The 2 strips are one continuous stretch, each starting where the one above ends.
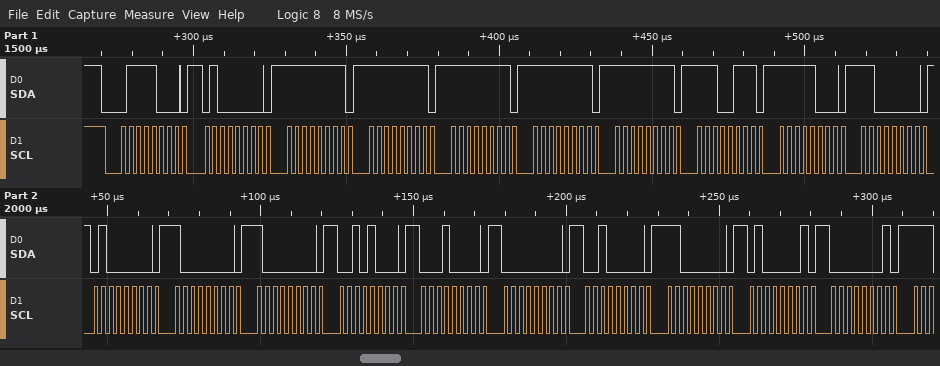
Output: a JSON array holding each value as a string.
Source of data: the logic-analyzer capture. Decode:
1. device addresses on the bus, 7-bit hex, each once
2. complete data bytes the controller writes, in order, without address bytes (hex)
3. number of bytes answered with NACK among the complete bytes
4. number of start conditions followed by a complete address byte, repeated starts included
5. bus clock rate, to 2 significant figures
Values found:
["0x3C", "40 FF FF FF FF FF E7 F8 C0 40 80 80 28 10 00 20 C0 41 01", "0", "1", "400 kHz"]
